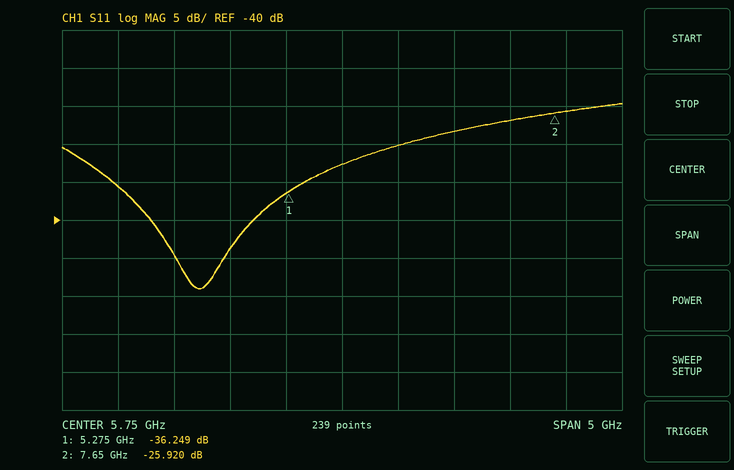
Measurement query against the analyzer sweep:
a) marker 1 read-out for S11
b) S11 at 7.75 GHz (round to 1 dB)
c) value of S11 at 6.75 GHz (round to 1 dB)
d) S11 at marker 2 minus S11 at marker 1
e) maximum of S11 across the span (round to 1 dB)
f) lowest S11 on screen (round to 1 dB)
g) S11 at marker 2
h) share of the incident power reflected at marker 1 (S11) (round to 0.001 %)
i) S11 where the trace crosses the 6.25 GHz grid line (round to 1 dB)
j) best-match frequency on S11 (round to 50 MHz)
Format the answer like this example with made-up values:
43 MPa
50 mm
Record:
-36.249 dB
-26 dB
-28 dB
10.329 dB
-25 dB
-49 dB
-25.920 dB
0.024 %
-30 dB
4.45 GHz
